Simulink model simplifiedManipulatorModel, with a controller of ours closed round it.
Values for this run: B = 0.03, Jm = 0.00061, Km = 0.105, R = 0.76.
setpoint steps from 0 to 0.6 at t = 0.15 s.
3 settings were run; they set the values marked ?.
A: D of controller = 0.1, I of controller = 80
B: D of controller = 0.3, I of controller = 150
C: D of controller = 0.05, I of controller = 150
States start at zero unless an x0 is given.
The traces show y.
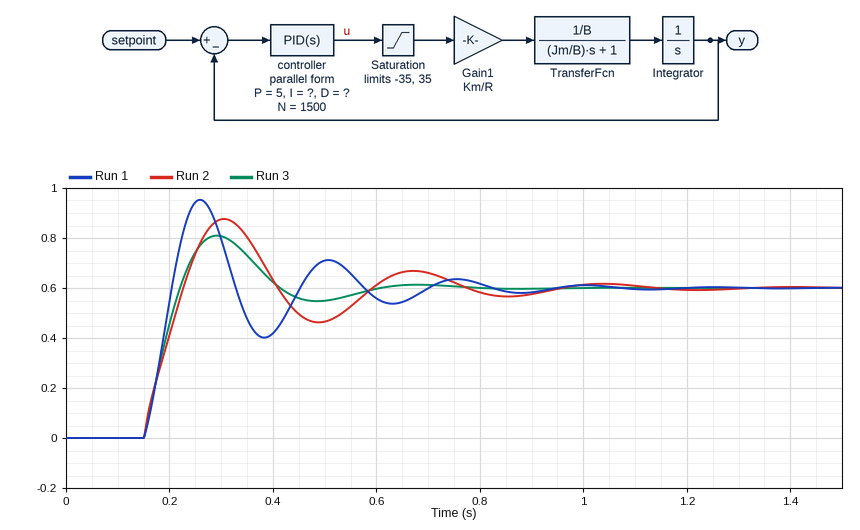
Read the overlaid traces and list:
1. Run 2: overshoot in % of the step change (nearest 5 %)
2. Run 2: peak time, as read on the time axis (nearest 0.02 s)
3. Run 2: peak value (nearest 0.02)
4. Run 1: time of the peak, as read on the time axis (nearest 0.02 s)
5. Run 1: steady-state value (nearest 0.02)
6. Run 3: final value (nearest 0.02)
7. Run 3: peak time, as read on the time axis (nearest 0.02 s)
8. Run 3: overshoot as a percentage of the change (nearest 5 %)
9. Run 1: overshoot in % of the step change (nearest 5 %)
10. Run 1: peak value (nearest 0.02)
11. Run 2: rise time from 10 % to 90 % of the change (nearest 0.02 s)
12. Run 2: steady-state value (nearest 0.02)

45 %
0.30 s
0.88
0.26 s
0.60
0.60
0.30 s
35 %
60 %
0.96
0.06 s
0.60
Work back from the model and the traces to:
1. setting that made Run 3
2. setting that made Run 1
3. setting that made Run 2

A
C
B
